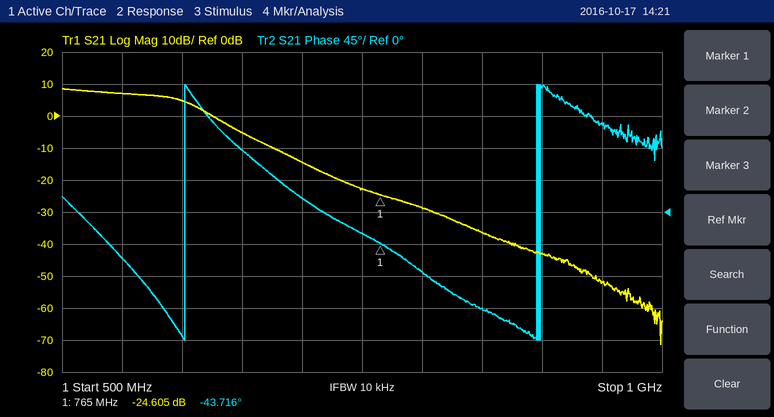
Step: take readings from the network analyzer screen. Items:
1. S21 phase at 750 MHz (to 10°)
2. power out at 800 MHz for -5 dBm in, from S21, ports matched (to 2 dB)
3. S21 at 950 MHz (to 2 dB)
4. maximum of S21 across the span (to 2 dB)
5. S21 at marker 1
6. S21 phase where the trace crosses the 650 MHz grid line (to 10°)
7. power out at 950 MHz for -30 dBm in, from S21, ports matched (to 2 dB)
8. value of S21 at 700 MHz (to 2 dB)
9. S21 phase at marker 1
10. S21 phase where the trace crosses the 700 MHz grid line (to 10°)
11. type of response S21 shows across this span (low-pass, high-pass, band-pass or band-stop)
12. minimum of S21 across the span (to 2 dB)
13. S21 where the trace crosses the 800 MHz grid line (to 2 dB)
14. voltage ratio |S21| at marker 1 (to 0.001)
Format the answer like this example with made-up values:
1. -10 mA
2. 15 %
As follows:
1. -30°
2. -34 dBm
3. -52 dB
4. 8 dB
5. -24.605 dB
6. 90°
7. -82 dBm
8. -14 dB
9. -43.716°
10. 20°
11. low-pass
12. -72 dB
13. -28 dB
14. 0.059
